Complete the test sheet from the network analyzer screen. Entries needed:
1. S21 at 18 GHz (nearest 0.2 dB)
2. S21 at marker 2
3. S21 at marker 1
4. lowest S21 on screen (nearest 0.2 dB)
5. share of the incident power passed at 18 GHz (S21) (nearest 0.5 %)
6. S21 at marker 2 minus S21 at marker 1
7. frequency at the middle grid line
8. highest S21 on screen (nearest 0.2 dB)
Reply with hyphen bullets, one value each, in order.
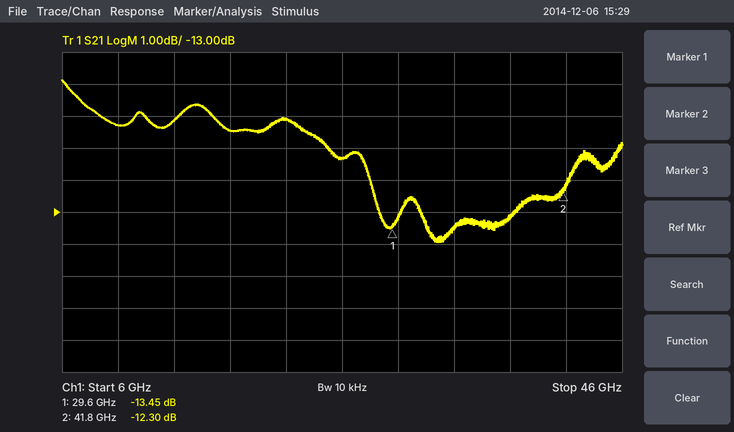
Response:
- -10.4 dB
- -12.30 dB
- -13.45 dB
- -14.0 dB
- 9.0 %
- 1.15 dB
- 26 GHz
- -8.8 dB
